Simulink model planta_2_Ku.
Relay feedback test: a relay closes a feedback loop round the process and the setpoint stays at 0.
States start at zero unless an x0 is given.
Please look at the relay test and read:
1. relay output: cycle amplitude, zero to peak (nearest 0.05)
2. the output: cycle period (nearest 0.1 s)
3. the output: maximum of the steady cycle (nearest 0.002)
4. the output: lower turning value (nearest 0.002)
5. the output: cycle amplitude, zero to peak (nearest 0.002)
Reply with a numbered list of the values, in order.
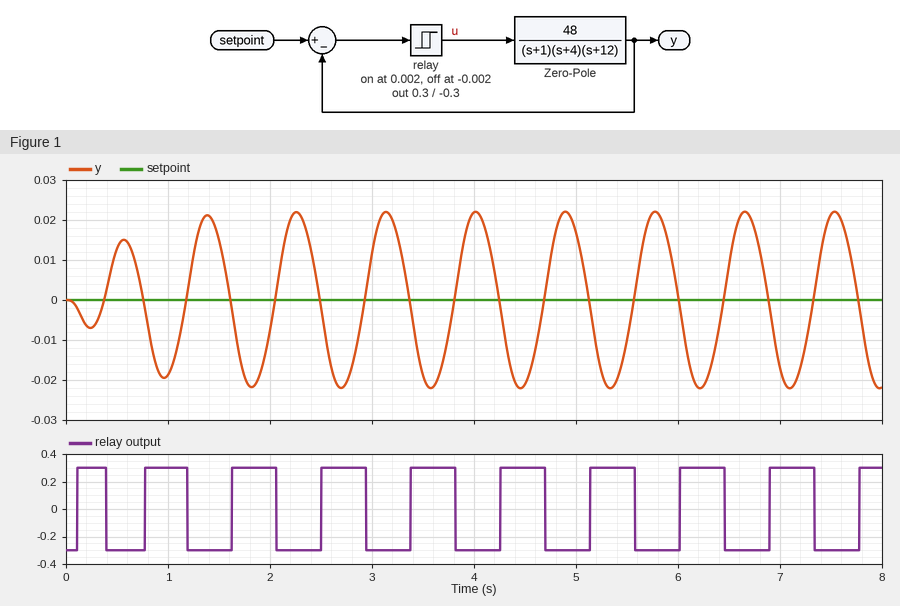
1. 0.30
2. 0.9 s
3. 0.022
4. -0.022
5. 0.022
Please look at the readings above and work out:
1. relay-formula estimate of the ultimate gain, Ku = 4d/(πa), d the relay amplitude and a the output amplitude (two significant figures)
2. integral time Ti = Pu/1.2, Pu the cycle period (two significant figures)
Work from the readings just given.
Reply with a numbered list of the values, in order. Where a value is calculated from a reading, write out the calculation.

1. 4 × 0.3 / (π × 0.022) = 17
2. 0.9 / 1.2 = 0.75 s
